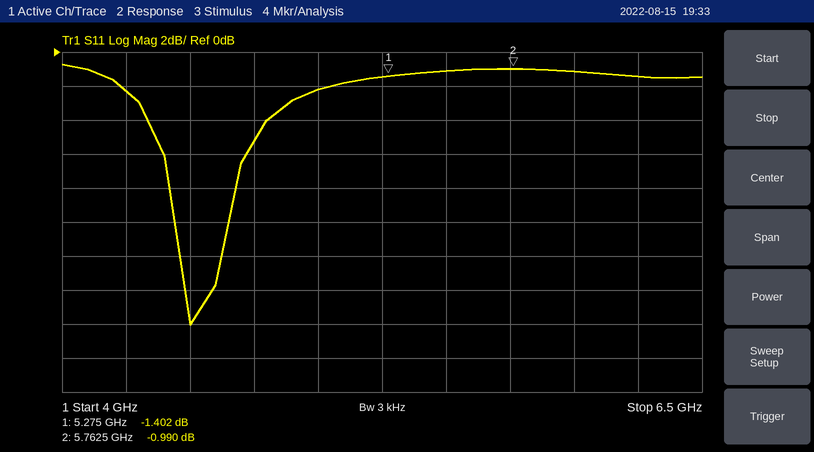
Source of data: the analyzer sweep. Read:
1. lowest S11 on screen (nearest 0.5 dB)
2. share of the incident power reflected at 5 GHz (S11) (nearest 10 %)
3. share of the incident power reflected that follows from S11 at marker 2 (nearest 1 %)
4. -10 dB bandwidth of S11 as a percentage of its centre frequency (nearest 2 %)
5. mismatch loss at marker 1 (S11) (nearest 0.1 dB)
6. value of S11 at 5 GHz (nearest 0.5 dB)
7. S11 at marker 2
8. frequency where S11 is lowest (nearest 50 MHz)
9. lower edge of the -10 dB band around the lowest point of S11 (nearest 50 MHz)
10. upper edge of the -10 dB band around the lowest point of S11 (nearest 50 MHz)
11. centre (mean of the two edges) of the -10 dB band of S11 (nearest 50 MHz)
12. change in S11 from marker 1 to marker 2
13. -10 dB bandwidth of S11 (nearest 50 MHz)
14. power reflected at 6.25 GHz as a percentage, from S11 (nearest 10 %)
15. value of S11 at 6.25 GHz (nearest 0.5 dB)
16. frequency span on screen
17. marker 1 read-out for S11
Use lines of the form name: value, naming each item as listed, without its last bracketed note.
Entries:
lowest S11 on screen: -16.0 dB
share of the incident power reflected at 5 GHz (S11): 60 %
share of the incident power reflected that follows from S11 at marker 2: 80 %
-10 dB bandwidth of S11 as a percentage of its centre frequency: 4 %
mismatch loss at marker 1 (S11): 5.6 dB
value of S11 at 5 GHz: -2.0 dB
S11 at marker 2: -0.990 dB
frequency where S11 is lowest: 4.50 GHz
lower edge of the -10 dB band around the lowest point of S11: 4.45 GHz
upper edge of the -10 dB band around the lowest point of S11: 4.65 GHz
centre (mean of the two edges) of the -10 dB band of S11: 4.55 GHz
change in S11 from marker 1 to marker 2: 0.412 dB
-10 dB bandwidth of S11: 200 MHz
power reflected at 6.25 GHz as a percentage, from S11: 70 %
value of S11 at 6.25 GHz: -1.5 dB
frequency span on screen: 2.5 GHz
marker 1 read-out for S11: -1.402 dB
